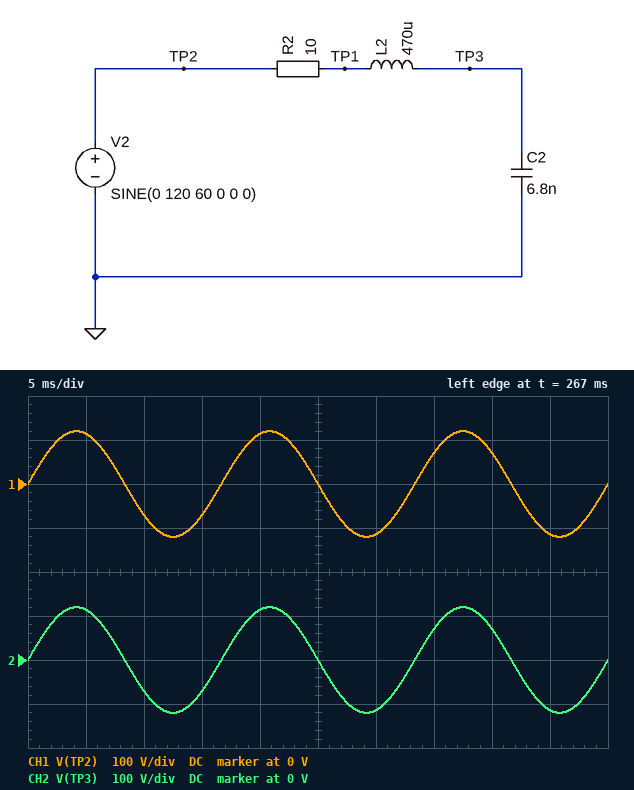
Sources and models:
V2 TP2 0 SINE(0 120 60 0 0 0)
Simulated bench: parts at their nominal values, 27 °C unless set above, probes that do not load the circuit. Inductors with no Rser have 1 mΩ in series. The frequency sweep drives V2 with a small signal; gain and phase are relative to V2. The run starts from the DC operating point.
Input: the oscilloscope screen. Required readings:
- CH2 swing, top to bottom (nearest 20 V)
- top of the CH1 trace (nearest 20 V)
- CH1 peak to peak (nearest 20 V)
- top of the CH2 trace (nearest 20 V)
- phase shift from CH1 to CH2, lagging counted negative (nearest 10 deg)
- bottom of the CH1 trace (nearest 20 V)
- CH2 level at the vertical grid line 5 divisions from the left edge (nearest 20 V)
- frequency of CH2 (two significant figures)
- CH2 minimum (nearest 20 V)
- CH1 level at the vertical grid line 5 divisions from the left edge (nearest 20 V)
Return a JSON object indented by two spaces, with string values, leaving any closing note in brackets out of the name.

{
  "CH2 swing, top to bottom": "240 V",
  "top of the CH1 trace": "120 V",
  "CH1 peak to peak": "240 V",
  "top of the CH2 trace": "120 V",
  "phase shift from CH1 to CH2, lagging counted negative": "0 deg",
  "bottom of the CH1 trace": "-120 V",
  "CH2 level at the vertical grid line 5 divisions from the left edge": "0 V",
  "frequency of CH2": "60 Hz",
  "CH2 minimum": "-120 V",
  "CH1 level at the vertical grid line 5 divisions from the left edge": "0 V"
}
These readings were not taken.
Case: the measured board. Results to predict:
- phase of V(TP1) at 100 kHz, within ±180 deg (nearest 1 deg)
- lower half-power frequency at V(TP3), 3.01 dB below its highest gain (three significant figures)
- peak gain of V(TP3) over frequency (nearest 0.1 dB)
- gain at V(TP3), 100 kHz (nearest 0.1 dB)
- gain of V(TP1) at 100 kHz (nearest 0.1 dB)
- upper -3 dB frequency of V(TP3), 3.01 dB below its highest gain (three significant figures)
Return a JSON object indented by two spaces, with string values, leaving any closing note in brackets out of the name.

{
  "phase of V(TP1) at 100 kHz, within ±180 deg": "9 deg",
  "lower half-power frequency at V(TP3), 3.01 dB below its highest gain": "87.3 kHz",
  "peak gain of V(TP3) over frequency": "28.4 dB",
  "gain at V(TP3), 100 kHz": "11.5 dB",
  "gain of V(TP1) at 100 kHz": "-0.1 dB",
  "upper -3 dB frequency of V(TP3), 3.01 dB below its highest gain": "90.7 kHz"
}
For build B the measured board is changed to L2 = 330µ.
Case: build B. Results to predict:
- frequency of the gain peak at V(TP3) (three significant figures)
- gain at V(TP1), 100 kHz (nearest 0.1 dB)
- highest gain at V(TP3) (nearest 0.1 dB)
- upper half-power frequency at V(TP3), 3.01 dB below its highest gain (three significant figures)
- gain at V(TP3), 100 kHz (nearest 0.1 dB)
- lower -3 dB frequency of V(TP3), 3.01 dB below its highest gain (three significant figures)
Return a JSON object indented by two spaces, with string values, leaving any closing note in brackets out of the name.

{
  "frequency of the gain peak at V(TP3)": "106 kHz",
  "gain at V(TP1), 100 kHz": "-0.6 dB",
  "highest gain at V(TP3)": "26.9 dB",
  "upper half-power frequency at V(TP3), 3.01 dB below its highest gain": "109 kHz",
  "gain at V(TP3), 100 kHz": "18.3 dB",
  "lower -3 dB frequency of V(TP3), 3.01 dB below its highest gain": "104 kHz"
}
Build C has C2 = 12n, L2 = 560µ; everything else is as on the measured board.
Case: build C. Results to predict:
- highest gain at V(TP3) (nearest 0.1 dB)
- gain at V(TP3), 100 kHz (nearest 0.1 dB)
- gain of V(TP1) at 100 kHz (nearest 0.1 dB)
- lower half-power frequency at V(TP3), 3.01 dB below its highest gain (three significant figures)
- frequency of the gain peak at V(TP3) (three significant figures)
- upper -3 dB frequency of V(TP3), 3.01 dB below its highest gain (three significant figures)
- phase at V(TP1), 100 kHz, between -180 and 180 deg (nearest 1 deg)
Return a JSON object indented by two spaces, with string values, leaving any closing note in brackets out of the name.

{
  "highest gain at V(TP3)": "26.7 dB",
  "gain at V(TP3), 100 kHz": "-4.4 dB",
  "gain of V(TP1) at 100 kHz": "0 dB",
  "lower half-power frequency at V(TP3), 3.01 dB below its highest gain": "59.9 kHz",
  "frequency of the gain peak at V(TP3)": "61.4 kHz",
  "upper -3 dB frequency of V(TP3), 3.01 dB below its highest gain": "62.8 kHz",
  "phase at V(TP1), 100 kHz, between -180 and 180 deg": "3 deg"
}
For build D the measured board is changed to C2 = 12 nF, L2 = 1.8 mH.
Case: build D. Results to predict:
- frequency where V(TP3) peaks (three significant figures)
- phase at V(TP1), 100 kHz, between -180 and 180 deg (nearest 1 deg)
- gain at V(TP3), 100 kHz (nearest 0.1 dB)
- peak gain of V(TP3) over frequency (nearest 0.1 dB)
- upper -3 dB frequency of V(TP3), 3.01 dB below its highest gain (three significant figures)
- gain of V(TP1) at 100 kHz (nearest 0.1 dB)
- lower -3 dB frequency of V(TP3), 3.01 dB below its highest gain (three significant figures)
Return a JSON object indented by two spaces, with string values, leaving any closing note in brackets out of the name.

{
  "frequency where V(TP3) peaks": "34.2 kHz",
  "phase at V(TP1), 100 kHz, between -180 and 180 deg": "1 deg",
  "gain at V(TP3), 100 kHz": "-17.5 dB",
  "peak gain of V(TP3) over frequency": "31.8 dB",
  "upper -3 dB frequency of V(TP3), 3.01 dB below its highest gain": "34.7 kHz",
  "gain of V(TP1) at 100 kHz": "0 dB",
  "lower -3 dB frequency of V(TP3), 3.01 dB below its highest gain": "33.8 kHz"
}
